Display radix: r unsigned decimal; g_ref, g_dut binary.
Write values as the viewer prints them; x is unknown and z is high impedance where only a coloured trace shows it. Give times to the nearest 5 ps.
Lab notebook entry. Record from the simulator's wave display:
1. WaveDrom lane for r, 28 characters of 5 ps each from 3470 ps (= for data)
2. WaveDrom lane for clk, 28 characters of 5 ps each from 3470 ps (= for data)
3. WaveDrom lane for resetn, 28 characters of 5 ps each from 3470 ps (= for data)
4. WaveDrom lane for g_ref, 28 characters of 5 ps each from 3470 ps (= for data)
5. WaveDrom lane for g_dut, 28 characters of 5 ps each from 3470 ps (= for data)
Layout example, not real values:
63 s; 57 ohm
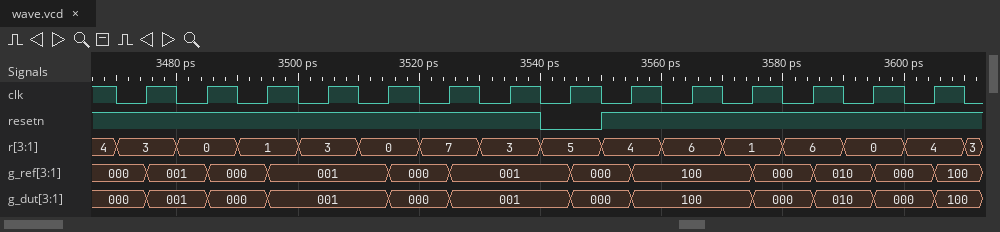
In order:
{name: 'r', wave: '=.=.=.=.=.=.=.=.=.=.=.=.=.=.', data: '3 0 1 3 0 7 3 5 4 6 1 6 0 4'}; {name: 'clk', wave: '0101010101010101010101010101'}; {name: 'resetn', wave: '1.............0.1...........'}; {name: 'g_ref', wave: '==.=.=...=.=...=.=...=.=.=.=', data: '000 001 000 001 000 001 000 100 000 010 000 100'}; {name: 'g_dut', wave: '==.=.=...=.=...=.=...=.=.=.=', data: '000 001 000 001 000 001 000 100 000 010 000 100'}
